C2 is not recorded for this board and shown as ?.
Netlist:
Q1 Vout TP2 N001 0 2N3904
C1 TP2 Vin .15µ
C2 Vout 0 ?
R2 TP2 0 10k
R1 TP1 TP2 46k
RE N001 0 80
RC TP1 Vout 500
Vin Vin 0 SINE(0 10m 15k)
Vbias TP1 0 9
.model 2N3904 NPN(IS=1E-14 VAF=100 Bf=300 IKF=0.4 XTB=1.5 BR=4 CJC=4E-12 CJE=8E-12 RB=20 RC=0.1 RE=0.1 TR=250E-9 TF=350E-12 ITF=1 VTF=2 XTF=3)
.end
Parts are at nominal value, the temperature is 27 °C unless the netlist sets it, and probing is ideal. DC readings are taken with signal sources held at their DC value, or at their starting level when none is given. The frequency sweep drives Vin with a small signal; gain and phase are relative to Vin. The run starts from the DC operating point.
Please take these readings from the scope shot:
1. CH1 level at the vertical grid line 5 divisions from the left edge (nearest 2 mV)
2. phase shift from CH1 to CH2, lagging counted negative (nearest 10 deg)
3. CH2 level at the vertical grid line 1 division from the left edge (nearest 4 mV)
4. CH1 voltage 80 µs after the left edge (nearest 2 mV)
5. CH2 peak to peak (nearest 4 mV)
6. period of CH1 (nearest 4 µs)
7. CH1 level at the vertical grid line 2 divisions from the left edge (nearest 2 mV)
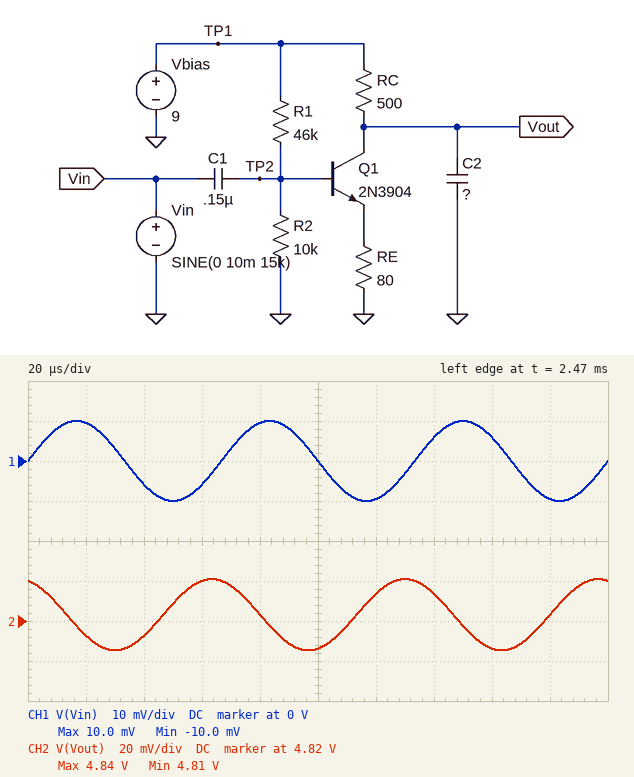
0 V
110 deg
4.812 V
10 mV
36 mV
68 µs
-6 mV
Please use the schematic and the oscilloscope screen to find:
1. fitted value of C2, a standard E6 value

68 nF
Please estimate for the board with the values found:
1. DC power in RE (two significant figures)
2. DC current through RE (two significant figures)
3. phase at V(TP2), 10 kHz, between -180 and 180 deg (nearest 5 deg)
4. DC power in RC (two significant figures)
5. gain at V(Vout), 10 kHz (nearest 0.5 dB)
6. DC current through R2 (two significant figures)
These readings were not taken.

5.6 mW
8.4 mA
0 deg
35 mW
8.0 dB
140 µA
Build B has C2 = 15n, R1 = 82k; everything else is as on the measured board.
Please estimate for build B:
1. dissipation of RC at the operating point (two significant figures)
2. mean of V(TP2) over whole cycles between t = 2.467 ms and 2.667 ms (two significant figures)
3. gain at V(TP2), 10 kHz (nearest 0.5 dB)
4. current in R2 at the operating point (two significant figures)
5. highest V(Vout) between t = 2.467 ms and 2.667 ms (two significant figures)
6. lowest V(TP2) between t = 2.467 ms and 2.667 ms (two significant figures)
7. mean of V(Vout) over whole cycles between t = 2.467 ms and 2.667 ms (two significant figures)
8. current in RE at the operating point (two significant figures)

3.8 mW
900 mV
0 dB
90 µA
7.7 V
890 mV
7.6 V
2.8 mA
